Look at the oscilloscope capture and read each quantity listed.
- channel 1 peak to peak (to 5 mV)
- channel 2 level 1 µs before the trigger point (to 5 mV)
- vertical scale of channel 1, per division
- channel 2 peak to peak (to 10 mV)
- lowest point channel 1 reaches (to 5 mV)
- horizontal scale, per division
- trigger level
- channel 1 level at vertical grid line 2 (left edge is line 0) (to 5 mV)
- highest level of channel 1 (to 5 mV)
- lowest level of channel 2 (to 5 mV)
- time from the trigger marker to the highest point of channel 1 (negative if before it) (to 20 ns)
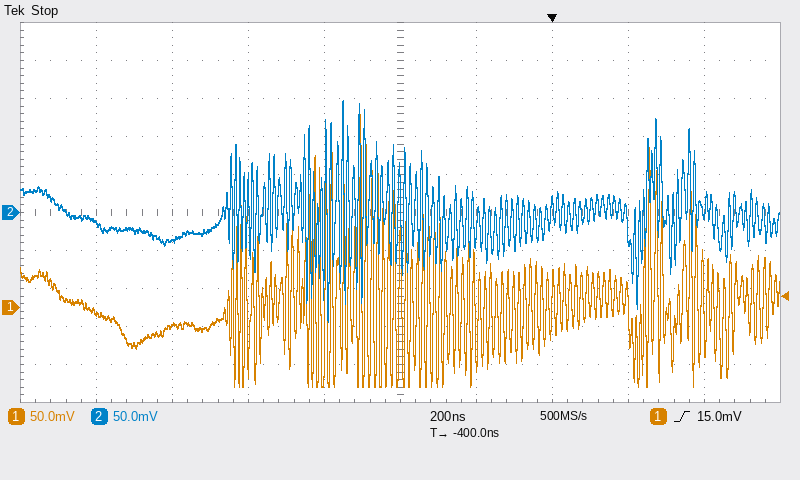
360 mV
-35 mV
50 mV
290 mV
-105 mV
200 ns
15.0 mV
-25 mV
255 mV
-145 mV
-500 ns
